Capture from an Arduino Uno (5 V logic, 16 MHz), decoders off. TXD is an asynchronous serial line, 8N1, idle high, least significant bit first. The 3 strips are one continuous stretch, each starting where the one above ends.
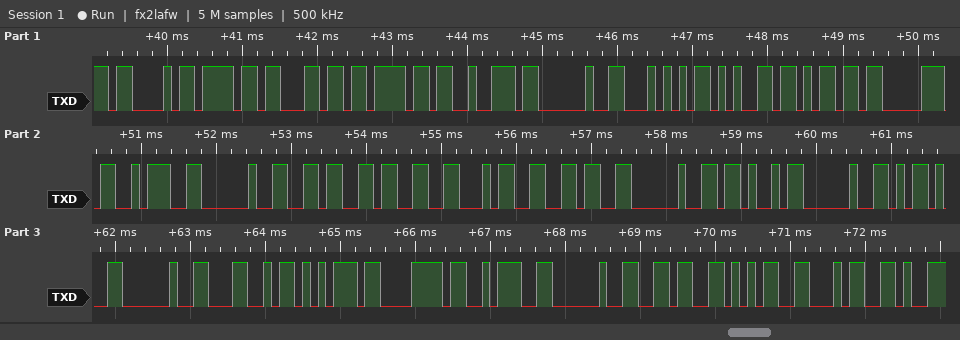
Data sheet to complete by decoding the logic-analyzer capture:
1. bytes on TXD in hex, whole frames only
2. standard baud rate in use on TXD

43 6F 6C 6F 72 20 54 65 6D 70 3A 20 36 33 34 36 20 4B 20 2D 20 4C 75 78 3A 20 36 35 34
9600 baud
